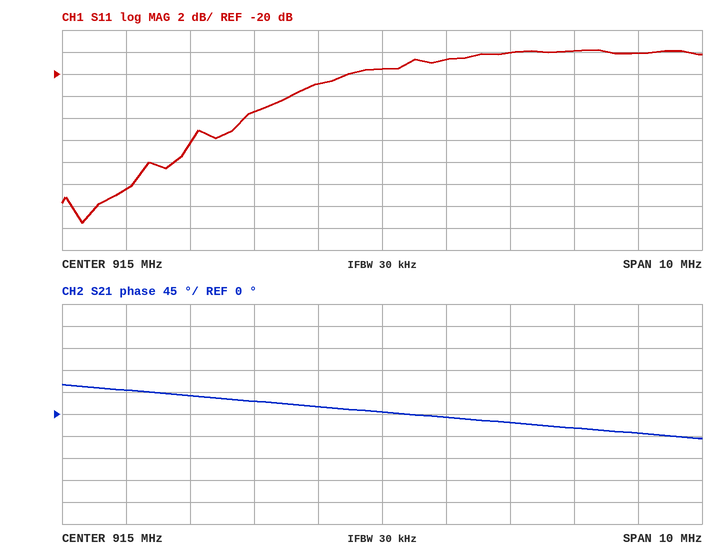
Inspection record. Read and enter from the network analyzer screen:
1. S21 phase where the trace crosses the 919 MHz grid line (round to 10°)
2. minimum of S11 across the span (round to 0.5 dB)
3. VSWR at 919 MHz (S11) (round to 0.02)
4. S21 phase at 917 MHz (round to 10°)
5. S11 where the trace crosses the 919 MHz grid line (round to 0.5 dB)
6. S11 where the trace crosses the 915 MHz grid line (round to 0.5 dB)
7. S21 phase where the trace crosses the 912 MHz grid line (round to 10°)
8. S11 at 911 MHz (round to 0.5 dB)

-40°
-33.5 dB
1.28
-20°
-18.0 dB
-19.5 dB
40°
-30.5 dB
